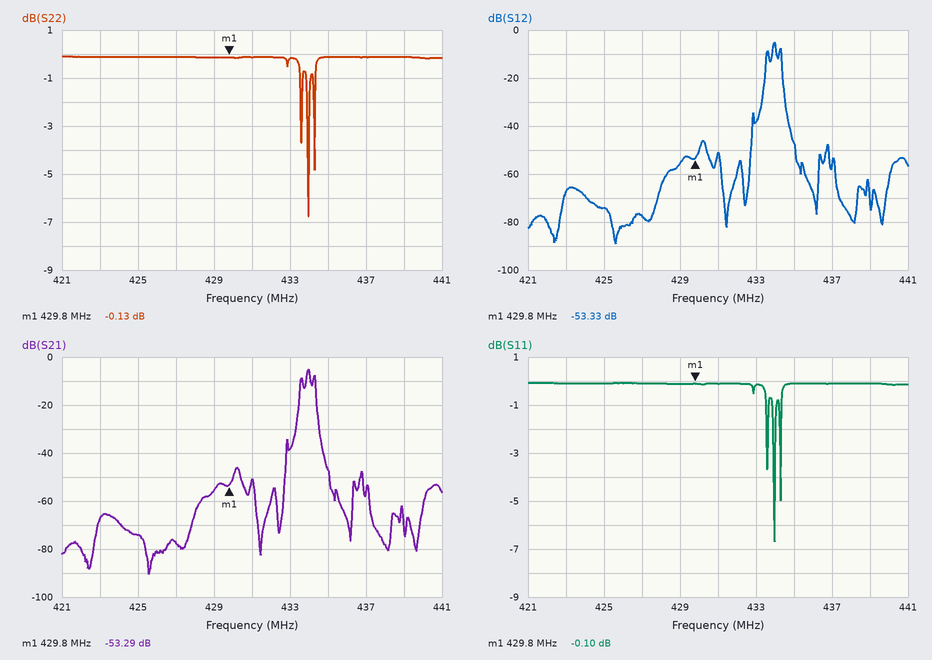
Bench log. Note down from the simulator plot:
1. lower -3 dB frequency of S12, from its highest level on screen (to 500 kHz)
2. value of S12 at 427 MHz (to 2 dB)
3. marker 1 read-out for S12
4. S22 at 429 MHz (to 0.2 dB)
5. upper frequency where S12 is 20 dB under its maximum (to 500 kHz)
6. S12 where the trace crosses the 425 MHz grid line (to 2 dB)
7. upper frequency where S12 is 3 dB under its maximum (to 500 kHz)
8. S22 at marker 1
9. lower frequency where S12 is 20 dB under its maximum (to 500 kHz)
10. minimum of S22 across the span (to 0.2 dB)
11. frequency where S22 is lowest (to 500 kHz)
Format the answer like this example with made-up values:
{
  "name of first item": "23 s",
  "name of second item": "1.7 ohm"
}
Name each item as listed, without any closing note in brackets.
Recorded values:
{
  "lower -3 dB frequency of S12, from its highest level on screen": "434.0 MHz",
  "value of S12 at 427 MHz": "-78 dB",
  "marker 1 read-out for S12": "-53.33 dB",
  "S22 at 429 MHz": "-0.2 dB",
  "upper frequency where S12 is 20 dB under its maximum": "434.5 MHz",
  "S12 where the trace crosses the 425 MHz grid line": "-74 dB",
  "upper frequency where S12 is 3 dB under its maximum": "434.0 MHz",
  "S22 at marker 1": "-0.13 dB",
  "lower frequency where S12 is 20 dB under its maximum": "433.5 MHz",
  "minimum of S22 across the span": "-6.8 dB",
  "frequency where S22 is lowest": "434.0 MHz"
}
